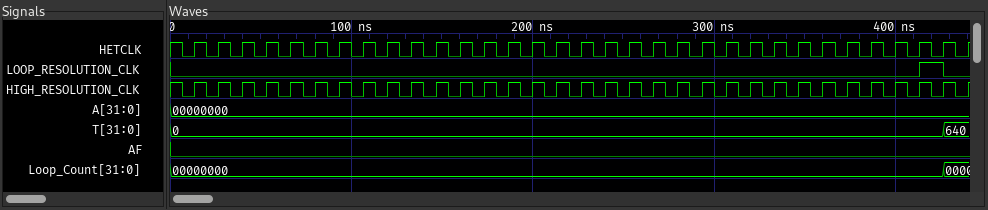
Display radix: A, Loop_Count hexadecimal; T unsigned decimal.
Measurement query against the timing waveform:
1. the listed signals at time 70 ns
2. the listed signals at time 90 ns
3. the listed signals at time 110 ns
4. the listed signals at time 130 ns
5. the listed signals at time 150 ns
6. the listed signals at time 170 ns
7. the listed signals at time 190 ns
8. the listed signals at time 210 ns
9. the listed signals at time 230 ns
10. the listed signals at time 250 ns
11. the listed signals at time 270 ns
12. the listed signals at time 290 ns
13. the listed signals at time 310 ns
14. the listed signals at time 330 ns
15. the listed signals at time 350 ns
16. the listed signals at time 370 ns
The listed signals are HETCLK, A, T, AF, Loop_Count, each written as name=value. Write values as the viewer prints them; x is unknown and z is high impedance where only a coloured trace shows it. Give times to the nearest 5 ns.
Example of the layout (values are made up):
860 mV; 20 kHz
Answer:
HETCLK=1, A=00000000, T=0, AF=0, Loop_Count=00000000; HETCLK=0, A=00000000, T=0, AF=0, Loop_Count=00000000; HETCLK=1, A=00000000, T=0, AF=0, Loop_Count=00000000; HETCLK=0, A=00000000, T=0, AF=0, Loop_Count=00000000; HETCLK=1, A=00000000, T=0, AF=0, Loop_Count=00000000; HETCLK=0, A=00000000, T=0, AF=0, Loop_Count=00000000; HETCLK=1, A=00000000, T=0, AF=0, Loop_Count=00000000; HETCLK=0, A=00000000, T=0, AF=0, Loop_Count=00000000; HETCLK=1, A=00000000, T=0, AF=0, Loop_Count=00000000; HETCLK=0, A=00000000, T=0, AF=0, Loop_Count=00000000; HETCLK=1, A=00000000, T=0, AF=0, Loop_Count=00000000; HETCLK=0, A=00000000, T=0, AF=0, Loop_Count=00000000; HETCLK=1, A=00000000, T=0, AF=0, Loop_Count=00000000; HETCLK=0, A=00000000, T=0, AF=0, Loop_Count=00000000; HETCLK=1, A=00000000, T=0, AF=0, Loop_Count=00000000; HETCLK=0, A=00000000, T=0, AF=0, Loop_Count=00000000
